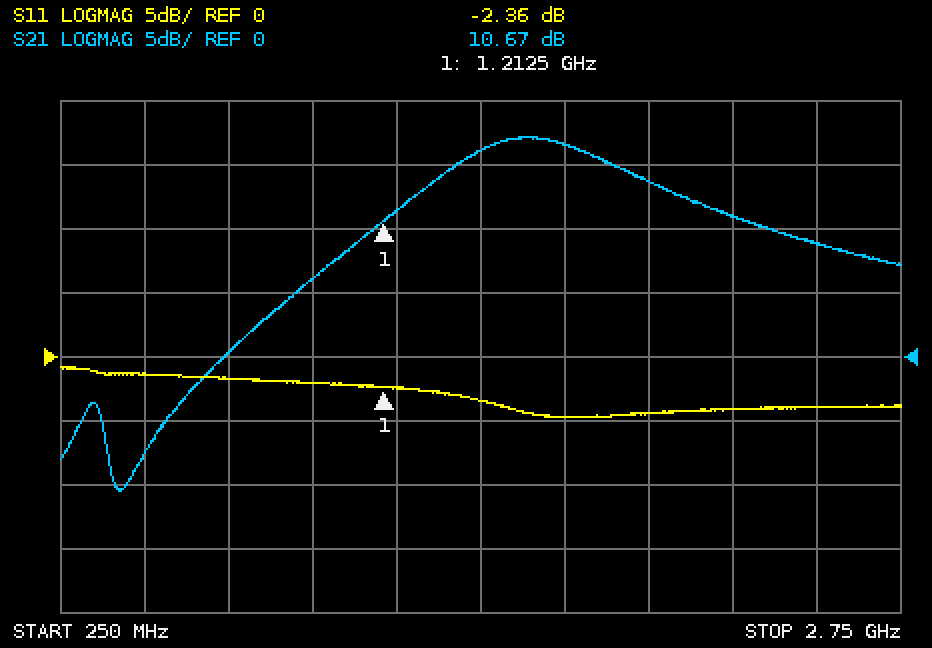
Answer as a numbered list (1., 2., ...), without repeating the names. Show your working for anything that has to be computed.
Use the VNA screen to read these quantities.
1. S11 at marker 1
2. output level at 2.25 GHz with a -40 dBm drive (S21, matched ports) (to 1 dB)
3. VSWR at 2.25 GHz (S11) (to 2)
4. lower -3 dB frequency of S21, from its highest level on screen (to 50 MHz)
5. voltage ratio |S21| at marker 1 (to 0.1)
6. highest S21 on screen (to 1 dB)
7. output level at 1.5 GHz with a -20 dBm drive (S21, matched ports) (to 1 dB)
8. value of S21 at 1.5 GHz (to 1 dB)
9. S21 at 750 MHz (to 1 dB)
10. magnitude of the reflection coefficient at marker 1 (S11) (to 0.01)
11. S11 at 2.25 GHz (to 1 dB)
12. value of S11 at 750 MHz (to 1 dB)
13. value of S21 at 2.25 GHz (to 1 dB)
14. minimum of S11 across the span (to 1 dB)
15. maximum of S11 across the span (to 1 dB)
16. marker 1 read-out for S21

1. -2.36 dB
2. -40 dBm + (11 dB) = -29 dBm
3. |Γ| = 10^(-4/20) = 0.6310; VSWR = (1 + 0.6310)/(1 − 0.6310) ≈ 4
4. 1.40 GHz
5. 10^(10.67/20) ≈ 3.4
6. 17 dB
7. -20 dBm + (16 dB) = -4 dBm
8. 16 dB
9. 0 dB
10. 10^(-2.36/20) ≈ 0.76
11. -4 dB
12. -2 dB
13. 11 dB
14. -5 dB
15. -1 dB
16. 10.67 dB
